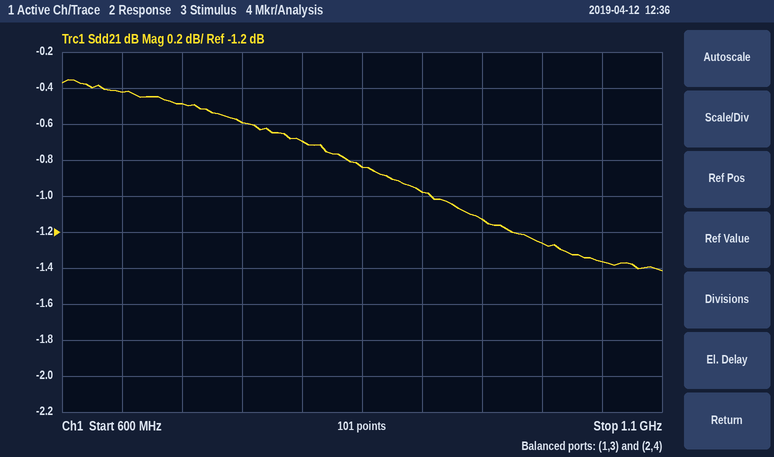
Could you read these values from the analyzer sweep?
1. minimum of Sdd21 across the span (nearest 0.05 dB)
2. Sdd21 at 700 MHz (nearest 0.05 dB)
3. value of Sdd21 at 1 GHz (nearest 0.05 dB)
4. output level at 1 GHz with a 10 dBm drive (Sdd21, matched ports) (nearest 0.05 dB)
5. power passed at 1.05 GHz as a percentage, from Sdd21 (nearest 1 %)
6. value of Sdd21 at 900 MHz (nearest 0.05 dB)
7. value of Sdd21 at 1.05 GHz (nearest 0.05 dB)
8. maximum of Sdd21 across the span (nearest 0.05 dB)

-1.40 dB
-0.50 dB
-1.25 dB
8.75 dBm
73 %
-1.00 dB
-1.35 dB
-0.35 dB
